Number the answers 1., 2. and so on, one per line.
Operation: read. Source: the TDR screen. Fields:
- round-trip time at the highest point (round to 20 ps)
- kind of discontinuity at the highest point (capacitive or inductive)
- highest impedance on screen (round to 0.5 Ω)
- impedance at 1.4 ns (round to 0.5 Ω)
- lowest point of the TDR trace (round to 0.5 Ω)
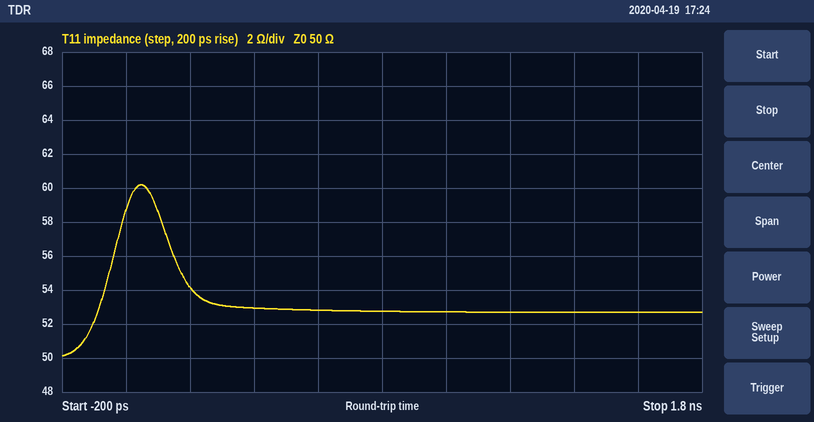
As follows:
1. 40 ps
2. inductive
3. 60.0 Ω
4. 52.5 Ω
5. 50.0 Ω
